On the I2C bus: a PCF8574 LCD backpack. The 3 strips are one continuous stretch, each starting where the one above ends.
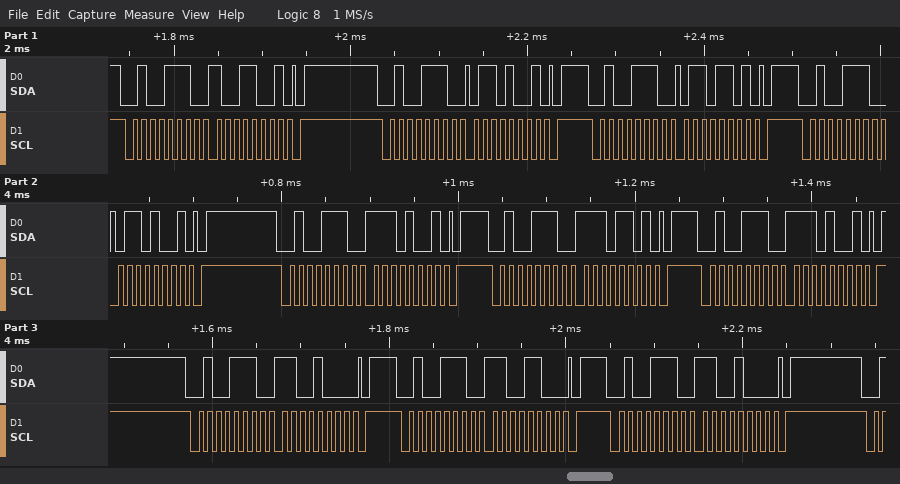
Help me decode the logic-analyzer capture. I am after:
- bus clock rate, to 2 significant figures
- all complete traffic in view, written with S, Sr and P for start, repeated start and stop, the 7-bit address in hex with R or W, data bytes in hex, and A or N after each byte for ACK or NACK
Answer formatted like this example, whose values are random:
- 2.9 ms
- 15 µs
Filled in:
- 100 kHz
- S 27W A 99 A P S 27W A 69 A P S 27W A 6D A P S 27W A 69 A P S 27W A E9 A P S 27W A ED A P S 27W A E9 A P S 27W A C8 A P S 27W A CC A P S 27W A C8 A P
